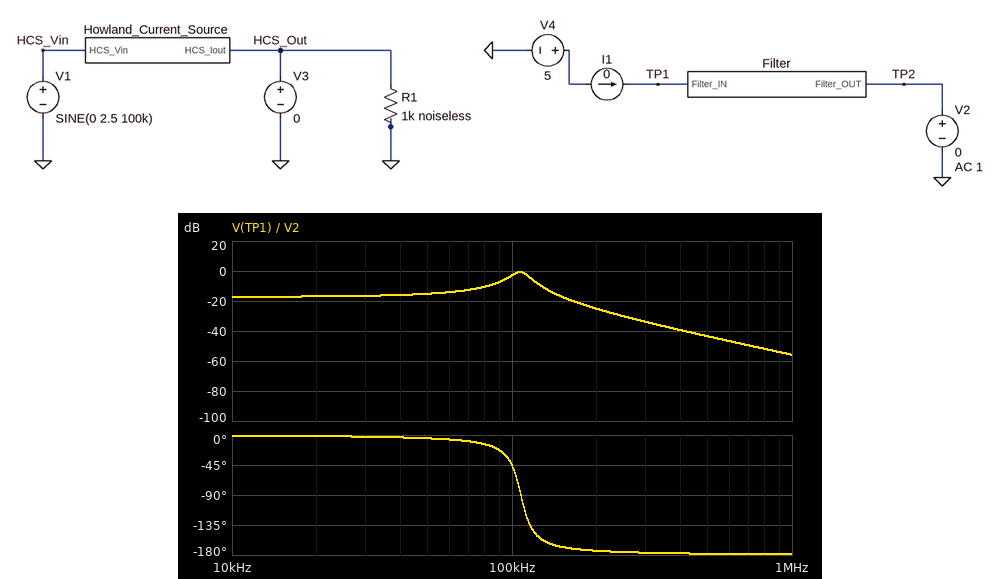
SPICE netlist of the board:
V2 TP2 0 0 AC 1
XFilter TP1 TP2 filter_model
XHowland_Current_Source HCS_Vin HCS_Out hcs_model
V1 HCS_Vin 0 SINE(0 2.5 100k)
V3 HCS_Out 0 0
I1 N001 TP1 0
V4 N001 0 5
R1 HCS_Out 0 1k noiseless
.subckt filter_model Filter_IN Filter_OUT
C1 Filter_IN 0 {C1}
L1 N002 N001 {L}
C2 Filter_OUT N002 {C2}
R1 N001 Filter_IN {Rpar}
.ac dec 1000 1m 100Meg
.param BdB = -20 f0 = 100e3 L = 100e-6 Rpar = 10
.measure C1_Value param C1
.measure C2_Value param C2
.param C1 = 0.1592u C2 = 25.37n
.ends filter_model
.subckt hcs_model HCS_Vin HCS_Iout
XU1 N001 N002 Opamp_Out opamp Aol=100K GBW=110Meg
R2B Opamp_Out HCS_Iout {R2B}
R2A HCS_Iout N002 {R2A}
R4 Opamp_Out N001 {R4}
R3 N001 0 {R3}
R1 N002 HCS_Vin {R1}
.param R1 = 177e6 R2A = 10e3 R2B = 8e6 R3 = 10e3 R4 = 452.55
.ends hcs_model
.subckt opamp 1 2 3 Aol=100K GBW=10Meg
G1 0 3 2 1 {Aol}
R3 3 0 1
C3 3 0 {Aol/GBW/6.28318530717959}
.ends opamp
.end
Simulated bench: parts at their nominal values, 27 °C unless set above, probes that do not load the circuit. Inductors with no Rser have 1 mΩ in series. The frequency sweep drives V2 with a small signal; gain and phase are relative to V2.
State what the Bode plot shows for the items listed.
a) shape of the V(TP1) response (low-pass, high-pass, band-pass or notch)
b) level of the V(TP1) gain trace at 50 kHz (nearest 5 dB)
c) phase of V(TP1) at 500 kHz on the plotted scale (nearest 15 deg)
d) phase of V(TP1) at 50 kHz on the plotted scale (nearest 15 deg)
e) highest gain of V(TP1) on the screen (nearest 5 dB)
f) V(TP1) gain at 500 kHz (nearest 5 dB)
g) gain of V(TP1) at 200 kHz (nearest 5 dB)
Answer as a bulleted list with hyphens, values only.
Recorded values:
- low-pass
- -15 dB
- -180 deg
- 0 deg
- 0 dB
- -45 dB
- -25 dB
